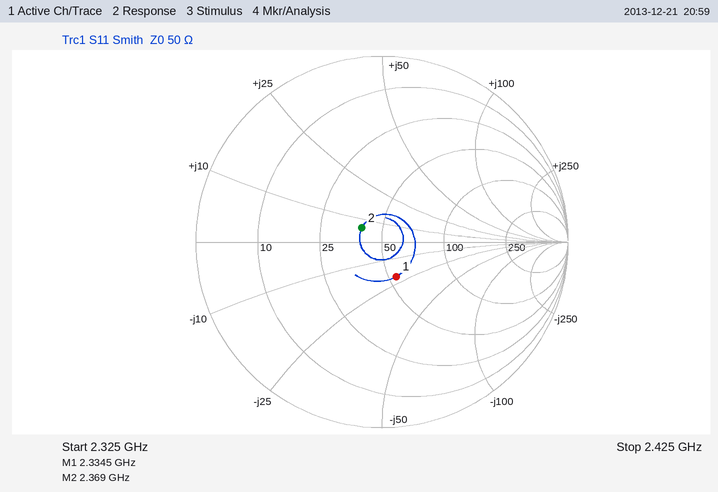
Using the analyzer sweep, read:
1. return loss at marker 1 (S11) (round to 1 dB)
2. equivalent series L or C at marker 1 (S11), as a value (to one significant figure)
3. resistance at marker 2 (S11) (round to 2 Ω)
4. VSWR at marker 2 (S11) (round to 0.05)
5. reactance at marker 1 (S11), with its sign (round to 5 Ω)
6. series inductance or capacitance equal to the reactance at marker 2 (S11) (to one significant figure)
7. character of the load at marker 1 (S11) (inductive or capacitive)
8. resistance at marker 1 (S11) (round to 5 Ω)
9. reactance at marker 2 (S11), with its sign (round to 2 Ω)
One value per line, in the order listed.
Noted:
14 dB
3 pF
40 Ω
1.30
-20 Ω
400 pH
capacitive
55 Ω
+6 Ω
